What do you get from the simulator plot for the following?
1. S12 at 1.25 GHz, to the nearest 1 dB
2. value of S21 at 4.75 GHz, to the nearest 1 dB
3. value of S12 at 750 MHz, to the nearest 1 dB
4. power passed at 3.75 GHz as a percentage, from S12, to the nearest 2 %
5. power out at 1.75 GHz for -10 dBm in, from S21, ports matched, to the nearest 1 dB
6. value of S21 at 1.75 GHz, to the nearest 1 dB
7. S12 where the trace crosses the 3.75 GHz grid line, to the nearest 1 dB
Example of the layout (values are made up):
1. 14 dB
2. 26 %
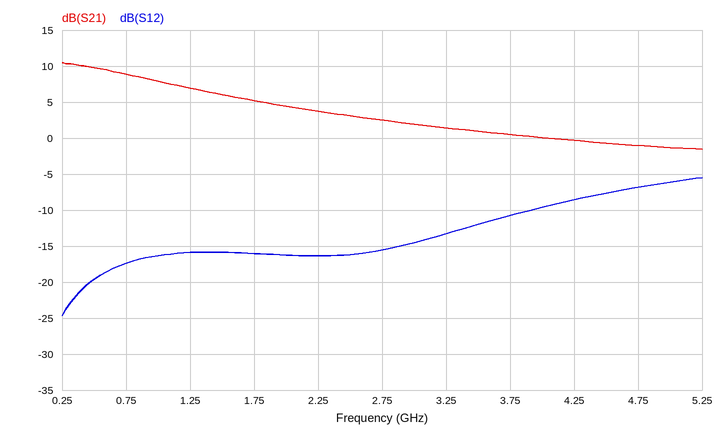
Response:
1. -16 dB
2. -1 dB
3. -17 dB
4. 8 %
5. -5 dBm
6. 5 dB
7. -11 dB
